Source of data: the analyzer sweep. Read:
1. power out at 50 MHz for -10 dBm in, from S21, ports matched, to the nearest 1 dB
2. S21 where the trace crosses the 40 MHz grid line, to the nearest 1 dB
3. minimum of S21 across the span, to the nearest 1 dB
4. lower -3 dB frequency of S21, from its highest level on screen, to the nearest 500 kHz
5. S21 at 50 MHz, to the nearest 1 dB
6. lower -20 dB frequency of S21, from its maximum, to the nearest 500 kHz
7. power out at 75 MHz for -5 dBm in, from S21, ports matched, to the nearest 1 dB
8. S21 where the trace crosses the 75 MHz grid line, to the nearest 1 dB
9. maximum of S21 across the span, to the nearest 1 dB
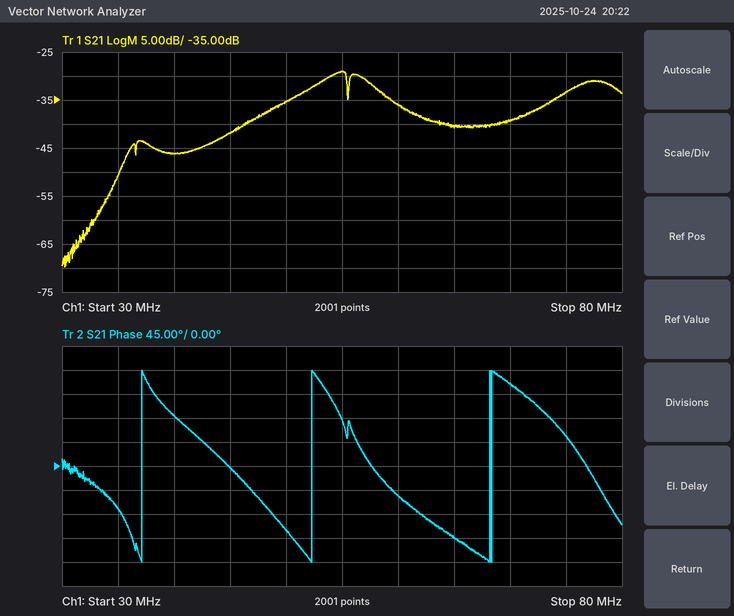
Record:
-45 dBm
-46 dB
-70 dB
52.5 MHz
-35 dB
35.5 MHz
-38 dBm
-33 dB
-29 dB
